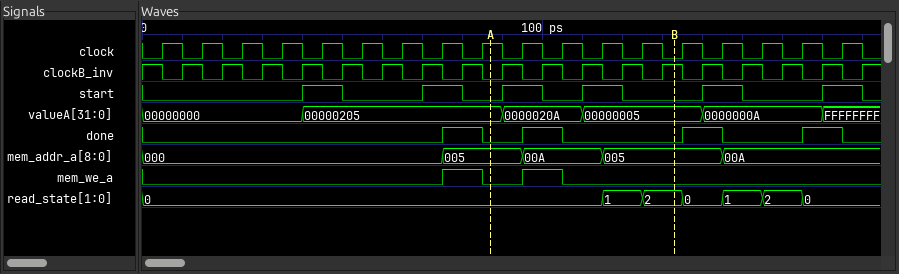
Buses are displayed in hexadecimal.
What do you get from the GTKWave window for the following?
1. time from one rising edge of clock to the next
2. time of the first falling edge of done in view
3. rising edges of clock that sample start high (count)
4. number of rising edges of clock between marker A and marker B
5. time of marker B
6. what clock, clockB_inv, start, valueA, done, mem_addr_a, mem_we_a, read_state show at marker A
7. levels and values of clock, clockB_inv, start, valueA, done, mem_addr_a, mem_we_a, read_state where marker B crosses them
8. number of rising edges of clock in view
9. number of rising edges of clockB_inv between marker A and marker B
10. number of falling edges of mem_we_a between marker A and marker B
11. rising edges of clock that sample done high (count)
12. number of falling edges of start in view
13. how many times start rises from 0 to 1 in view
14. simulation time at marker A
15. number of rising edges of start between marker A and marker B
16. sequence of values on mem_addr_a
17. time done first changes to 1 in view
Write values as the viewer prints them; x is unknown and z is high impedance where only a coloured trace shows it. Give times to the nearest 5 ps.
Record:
10 ps
85 ps
6
4
135 ps
clock=1, clockB_inv=0, start=0, valueA=00000205, done=0, mem_addr_a=005, mem_we_a=0, read_state=0
clock=0, clockB_inv=1, start=0, valueA=00000005, done=0, mem_addr_a=005, mem_we_a=0, read_state=2
18
5
1
4
6
6
85 ps
2
000, 005, 00A, 005, 00A
75 ps
